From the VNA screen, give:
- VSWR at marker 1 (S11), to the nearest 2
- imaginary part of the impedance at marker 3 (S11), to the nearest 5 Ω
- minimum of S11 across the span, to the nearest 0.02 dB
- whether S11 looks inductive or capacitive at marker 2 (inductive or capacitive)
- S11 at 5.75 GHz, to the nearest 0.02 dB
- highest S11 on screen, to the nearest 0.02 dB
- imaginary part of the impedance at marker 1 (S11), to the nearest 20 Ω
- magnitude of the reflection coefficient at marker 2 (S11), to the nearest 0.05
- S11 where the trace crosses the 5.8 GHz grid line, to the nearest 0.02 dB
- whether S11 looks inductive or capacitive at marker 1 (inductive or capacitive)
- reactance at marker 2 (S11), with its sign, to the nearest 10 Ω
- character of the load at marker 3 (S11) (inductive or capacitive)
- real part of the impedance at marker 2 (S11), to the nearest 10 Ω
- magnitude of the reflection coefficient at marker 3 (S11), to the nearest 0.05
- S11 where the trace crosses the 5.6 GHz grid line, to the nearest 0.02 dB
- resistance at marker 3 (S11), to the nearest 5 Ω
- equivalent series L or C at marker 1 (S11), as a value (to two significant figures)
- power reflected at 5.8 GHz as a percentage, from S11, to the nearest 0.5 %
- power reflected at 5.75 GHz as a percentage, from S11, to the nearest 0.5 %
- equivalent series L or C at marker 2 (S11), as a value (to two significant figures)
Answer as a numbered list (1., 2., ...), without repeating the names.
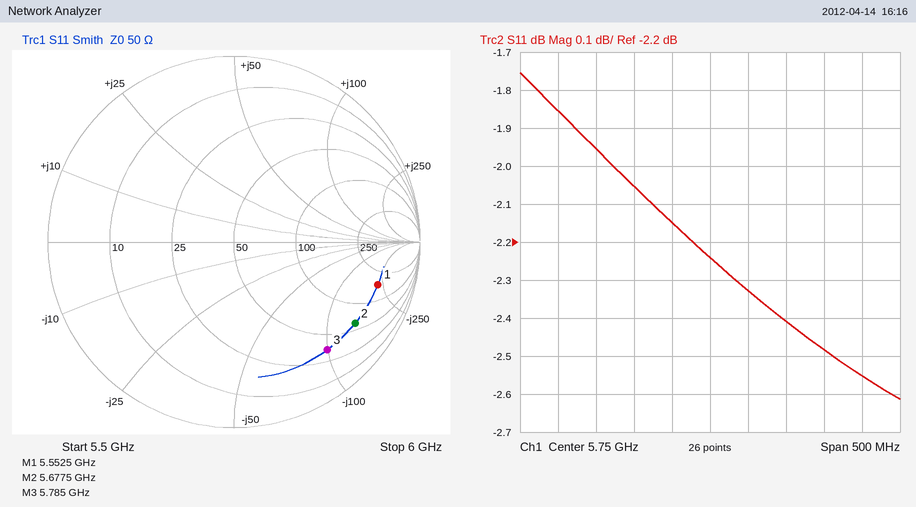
1. 10
2. -100 Ω
3. -2.62 dB
4. capacitive
5. -2.24 dB
6. -1.76 dB
7. -220 Ω
8. 0.80
9. -2.32 dB
10. capacitive
11. -140 Ω
12. capacitive
13. 60 Ω
14. 0.75
15. -1.96 dB
16. 35 Ω
17. 130 fF
18. 58.5 %
19. 59.5 %
20. 200 fF
